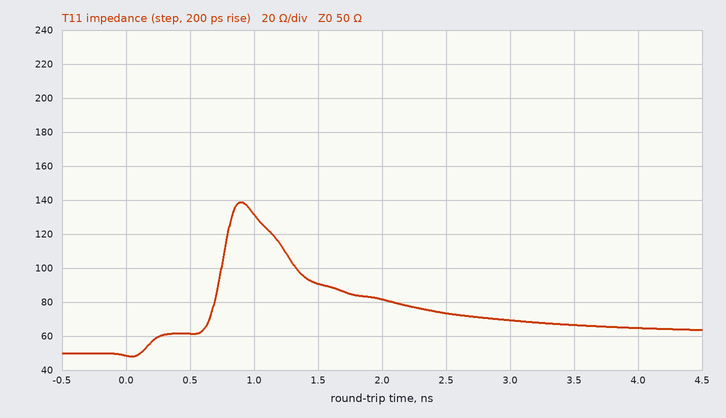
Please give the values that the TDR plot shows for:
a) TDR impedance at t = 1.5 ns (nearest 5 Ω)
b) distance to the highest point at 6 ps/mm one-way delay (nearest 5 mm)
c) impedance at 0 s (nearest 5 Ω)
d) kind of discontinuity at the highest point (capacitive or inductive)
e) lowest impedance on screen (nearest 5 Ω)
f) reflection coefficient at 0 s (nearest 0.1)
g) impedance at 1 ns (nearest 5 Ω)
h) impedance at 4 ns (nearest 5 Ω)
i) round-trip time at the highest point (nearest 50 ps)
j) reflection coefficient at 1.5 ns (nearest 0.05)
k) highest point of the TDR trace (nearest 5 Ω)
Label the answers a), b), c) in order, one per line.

a) 90 Ω
b) 75 mm
c) 50 Ω
d) inductive
e) 50 Ω
f) 0.0
g) 130 Ω
h) 65 Ω
i) 900 ps
j) +0.30
k) 140 Ω
